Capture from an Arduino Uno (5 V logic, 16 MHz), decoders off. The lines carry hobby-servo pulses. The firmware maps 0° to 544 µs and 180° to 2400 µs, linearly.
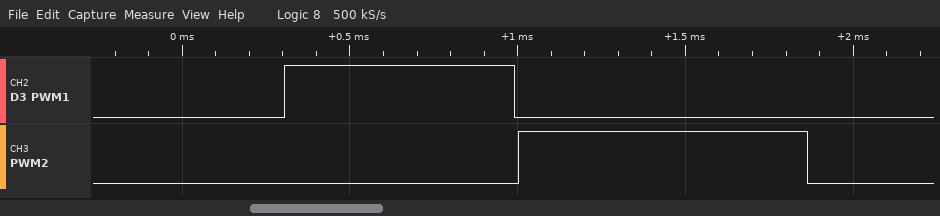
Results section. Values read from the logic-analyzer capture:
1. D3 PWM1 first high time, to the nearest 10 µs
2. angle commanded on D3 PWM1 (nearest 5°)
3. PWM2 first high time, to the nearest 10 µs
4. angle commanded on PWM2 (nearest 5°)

690 µs
15°
860 µs
30°
